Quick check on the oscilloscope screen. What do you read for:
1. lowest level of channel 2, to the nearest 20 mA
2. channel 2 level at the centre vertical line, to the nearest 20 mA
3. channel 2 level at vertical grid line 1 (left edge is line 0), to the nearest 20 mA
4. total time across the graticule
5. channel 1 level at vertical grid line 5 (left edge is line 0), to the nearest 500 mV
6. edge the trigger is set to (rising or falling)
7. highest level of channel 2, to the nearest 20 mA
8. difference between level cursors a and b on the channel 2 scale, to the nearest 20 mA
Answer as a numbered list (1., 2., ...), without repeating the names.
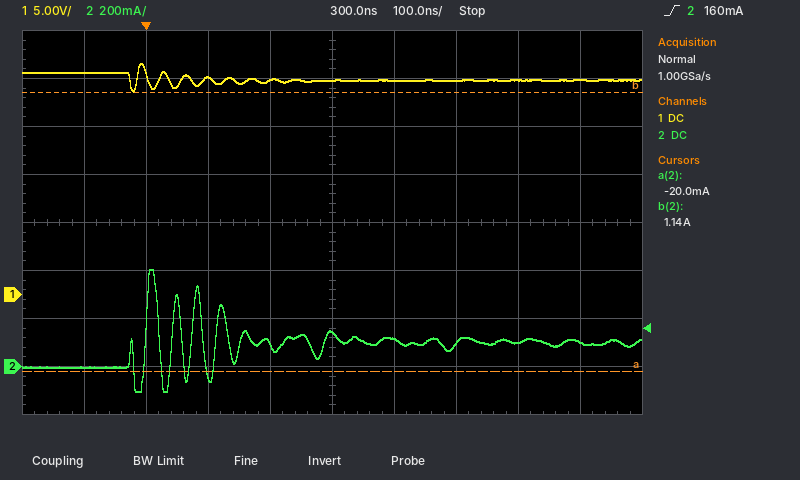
1. -100 mA
2. 140 mA
3. 0 mA
4. 1 µs
5. 22.5 V
6. rising
7. 400 mA
8. 1.16 A
